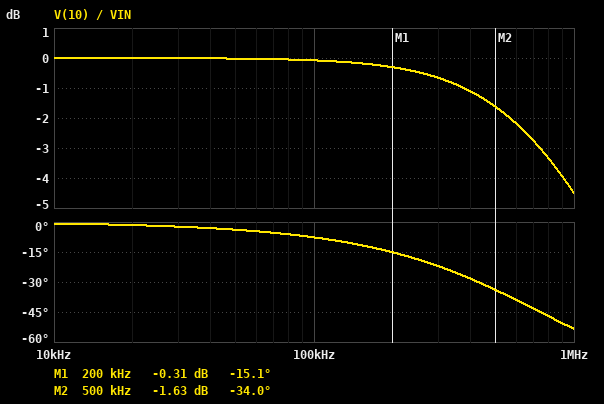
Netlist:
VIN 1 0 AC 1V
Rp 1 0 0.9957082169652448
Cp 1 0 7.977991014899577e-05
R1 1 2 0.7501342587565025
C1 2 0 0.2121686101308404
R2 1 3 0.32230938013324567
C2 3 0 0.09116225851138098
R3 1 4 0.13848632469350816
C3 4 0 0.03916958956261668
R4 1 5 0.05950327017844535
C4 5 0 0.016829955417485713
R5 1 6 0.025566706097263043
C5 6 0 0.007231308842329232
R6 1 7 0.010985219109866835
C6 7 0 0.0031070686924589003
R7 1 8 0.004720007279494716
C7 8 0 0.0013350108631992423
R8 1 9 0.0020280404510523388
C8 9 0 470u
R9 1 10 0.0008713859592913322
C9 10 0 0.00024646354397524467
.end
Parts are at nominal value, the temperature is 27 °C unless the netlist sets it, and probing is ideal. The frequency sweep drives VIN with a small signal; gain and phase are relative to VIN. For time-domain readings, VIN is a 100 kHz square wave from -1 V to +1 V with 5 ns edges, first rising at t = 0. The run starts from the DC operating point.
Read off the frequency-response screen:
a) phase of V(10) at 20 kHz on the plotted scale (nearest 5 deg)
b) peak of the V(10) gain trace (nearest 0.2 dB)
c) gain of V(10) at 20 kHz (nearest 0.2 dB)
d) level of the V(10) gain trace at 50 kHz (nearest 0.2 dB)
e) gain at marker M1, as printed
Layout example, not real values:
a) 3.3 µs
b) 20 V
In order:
a) 0 deg
b) 0 dB
c) 0 dB
d) 0 dB
e) -0.31 dB
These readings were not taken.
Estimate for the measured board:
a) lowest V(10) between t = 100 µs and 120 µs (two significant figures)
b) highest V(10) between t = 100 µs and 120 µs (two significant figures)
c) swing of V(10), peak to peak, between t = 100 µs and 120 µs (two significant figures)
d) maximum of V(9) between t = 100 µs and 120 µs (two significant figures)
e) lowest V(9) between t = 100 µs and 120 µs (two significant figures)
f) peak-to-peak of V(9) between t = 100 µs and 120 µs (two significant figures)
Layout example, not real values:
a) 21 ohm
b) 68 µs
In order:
a) -1.0 V
b) 1.0 V
c) 2.0 V
d) 990 mV
e) -990 mV
f) 2.0 V
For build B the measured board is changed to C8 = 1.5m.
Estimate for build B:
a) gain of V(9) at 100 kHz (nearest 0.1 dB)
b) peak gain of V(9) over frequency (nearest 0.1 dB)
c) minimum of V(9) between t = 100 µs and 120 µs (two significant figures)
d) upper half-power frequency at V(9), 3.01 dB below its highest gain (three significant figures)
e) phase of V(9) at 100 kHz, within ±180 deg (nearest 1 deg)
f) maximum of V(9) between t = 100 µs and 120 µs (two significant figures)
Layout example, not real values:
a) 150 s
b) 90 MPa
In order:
a) -6.7 dB
b) 0 dB
c) -680 mV
d) 52.3 kHz
e) -62 deg
f) 680 mV
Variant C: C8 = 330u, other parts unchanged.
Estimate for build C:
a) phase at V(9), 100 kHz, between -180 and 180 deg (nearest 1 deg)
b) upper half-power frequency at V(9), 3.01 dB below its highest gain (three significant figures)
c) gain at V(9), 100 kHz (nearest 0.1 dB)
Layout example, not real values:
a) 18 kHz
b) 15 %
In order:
a) -23 deg
b) 238 kHz
c) -0.7 dB
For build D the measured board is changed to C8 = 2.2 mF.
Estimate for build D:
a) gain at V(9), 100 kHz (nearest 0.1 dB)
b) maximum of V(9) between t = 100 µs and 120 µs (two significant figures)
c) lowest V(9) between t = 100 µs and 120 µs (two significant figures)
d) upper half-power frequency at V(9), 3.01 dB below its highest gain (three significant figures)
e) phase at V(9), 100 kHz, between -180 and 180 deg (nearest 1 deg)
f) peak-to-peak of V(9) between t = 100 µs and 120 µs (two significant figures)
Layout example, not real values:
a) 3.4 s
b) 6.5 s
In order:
a) -9.5 dB
b) 510 mV
c) -510 mV
d) 35.7 kHz
e) -70 deg
f) 1.0 V
